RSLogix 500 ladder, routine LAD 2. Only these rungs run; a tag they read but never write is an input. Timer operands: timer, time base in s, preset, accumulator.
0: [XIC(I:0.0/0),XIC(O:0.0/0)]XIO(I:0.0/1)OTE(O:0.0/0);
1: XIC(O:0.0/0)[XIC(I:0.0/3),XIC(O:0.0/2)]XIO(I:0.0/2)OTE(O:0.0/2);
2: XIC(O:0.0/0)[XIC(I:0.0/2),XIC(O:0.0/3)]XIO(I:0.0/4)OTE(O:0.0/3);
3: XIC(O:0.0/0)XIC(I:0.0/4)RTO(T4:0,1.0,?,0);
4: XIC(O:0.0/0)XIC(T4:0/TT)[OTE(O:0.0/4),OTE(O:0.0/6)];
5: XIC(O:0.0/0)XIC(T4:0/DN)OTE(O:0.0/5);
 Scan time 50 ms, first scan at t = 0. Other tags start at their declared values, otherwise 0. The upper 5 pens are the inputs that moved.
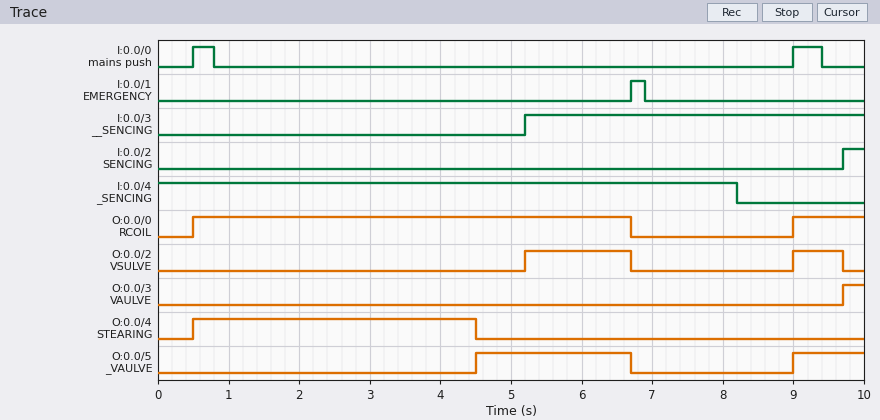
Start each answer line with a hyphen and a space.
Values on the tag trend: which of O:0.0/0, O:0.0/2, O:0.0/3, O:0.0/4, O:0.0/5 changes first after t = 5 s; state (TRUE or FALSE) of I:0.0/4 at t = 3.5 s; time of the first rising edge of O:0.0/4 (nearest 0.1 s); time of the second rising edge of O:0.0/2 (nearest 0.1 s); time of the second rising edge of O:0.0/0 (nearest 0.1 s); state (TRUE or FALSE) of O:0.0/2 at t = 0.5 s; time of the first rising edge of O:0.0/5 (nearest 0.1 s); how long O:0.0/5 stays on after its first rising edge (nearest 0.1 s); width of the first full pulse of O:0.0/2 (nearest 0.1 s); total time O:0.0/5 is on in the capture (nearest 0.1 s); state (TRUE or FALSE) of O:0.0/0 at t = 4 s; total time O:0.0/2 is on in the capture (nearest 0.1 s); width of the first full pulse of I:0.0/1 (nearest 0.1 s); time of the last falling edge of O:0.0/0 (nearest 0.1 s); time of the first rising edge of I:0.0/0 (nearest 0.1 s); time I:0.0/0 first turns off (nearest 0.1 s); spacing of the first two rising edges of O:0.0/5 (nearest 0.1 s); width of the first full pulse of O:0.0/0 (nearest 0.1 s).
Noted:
- O:0.0/2
- TRUE
- 0.5 s
- 9.0 s
- 9.0 s
- FALSE
- 4.5 s
- 2.2 s
- 1.5 s
- 3.2 s
- TRUE
- 2.2 s
- 0.2 s
- 6.7 s
- 0.5 s
- 0.8 s
- 4.5 s
- 6.2 s
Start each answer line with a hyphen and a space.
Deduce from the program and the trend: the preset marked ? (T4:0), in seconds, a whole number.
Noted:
- 4 s
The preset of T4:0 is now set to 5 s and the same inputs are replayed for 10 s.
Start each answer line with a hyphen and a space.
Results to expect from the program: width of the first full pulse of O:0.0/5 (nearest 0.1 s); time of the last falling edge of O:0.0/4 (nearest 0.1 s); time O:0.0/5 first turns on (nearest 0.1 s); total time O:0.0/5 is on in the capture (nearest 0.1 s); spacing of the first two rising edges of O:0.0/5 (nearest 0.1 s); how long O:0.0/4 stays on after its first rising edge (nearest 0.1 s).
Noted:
- 1.2 s
- 5.5 s
- 5.5 s
- 2.2 s
- 3.5 s
- 5.0 s
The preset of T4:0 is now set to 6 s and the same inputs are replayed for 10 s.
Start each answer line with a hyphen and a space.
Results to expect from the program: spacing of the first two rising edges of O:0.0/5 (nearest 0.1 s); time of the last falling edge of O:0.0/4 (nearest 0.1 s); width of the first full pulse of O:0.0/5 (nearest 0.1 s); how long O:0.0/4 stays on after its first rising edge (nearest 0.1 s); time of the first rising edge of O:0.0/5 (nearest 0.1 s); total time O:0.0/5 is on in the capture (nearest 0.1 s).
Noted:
- 2.5 s
- 6.5 s
- 0.2 s
- 6.0 s
- 6.5 s
- 1.2 s
